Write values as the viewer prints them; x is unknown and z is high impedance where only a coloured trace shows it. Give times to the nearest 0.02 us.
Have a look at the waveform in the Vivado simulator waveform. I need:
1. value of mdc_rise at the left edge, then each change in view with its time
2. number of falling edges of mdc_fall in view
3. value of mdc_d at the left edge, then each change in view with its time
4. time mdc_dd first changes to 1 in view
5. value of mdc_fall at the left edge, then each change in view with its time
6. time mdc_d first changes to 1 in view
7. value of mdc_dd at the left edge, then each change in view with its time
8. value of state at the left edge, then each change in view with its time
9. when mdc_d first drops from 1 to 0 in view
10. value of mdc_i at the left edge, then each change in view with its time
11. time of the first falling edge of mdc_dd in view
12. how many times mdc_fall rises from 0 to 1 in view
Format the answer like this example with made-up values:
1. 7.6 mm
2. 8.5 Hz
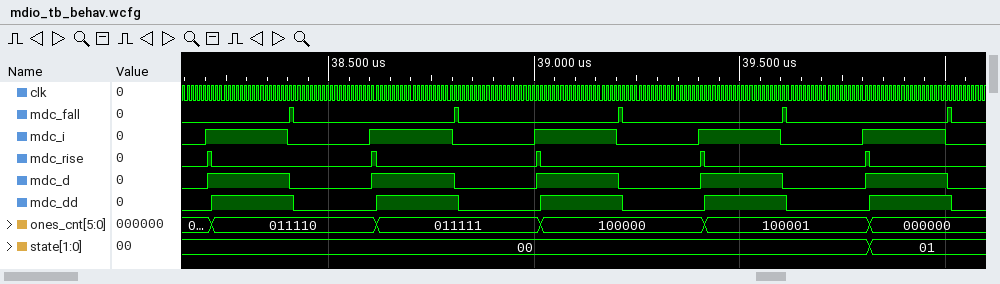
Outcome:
1. 0, 1 at 38.2 us, 0 at 38.22 us, 1 at 38.6 us, 0 at 38.62 us, 1 at 39 us, 0 at 39.02 us, 1 at 39.4 us, 0 at 39.42 us, 1 at 39.8 us, 0 at 39.82 us
2. 5
3. 0, 1 at 38.2 us, 0 at 38.4 us, 1 at 38.6 us, 0 at 38.8 us, 1 at 39 us, 0 at 39.2 us, 1 at 39.4 us, 0 at 39.6 us, 1 at 39.8 us, 0 at 40 us
4. 38.22 us
5. 0, 1 at 38.4 us, 0 at 38.42 us, 1 at 38.8 us, 0 at 38.82 us, 1 at 39.2 us, 0 at 39.22 us, 1 at 39.6 us, 0 at 39.62 us, 1 at 40 us, 0 at 40.02 us
6. 38.2 us
7. 0, 1 at 38.22 us, 0 at 38.42 us, 1 at 38.62 us, 0 at 38.82 us, 1 at 39.02 us, 0 at 39.22 us, 1 at 39.42 us, 0 at 39.62 us, 1 at 39.82 us, 0 at 40.02 us
8. 00, 01 at 39.82 us
9. 38.4 us
10. 0, 1 at 38.2 us, 0 at 38.4 us, 1 at 38.6 us, 0 at 38.8 us, 1 at 39 us, 0 at 39.2 us, 1 at 39.4 us, 0 at 39.6 us, 1 at 39.8 us, 0 at 40 us
11. 38.42 us
12. 5
